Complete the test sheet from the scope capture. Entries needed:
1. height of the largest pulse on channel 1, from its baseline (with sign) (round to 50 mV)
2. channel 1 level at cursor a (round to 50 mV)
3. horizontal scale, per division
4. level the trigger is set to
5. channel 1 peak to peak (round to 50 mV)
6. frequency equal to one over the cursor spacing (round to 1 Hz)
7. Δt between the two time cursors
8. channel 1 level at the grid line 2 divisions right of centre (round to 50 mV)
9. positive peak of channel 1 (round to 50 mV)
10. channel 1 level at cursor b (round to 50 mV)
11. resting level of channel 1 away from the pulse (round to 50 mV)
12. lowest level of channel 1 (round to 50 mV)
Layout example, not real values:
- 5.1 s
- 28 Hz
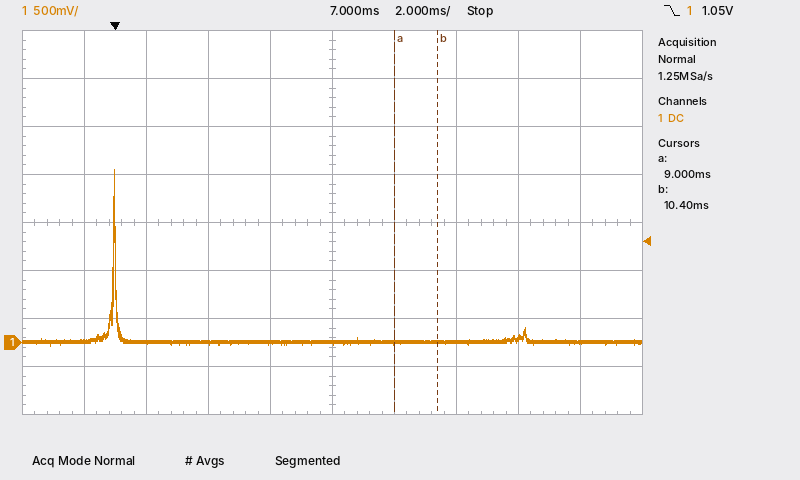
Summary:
- +1.80 V
- 0 mV
- 2 ms
- 1.05 V
- 1.85 V
- 714 Hz
- 1.4 ms
- 0 mV
- 1.80 V
- 0 mV
- 0 mV
- -50 mV
